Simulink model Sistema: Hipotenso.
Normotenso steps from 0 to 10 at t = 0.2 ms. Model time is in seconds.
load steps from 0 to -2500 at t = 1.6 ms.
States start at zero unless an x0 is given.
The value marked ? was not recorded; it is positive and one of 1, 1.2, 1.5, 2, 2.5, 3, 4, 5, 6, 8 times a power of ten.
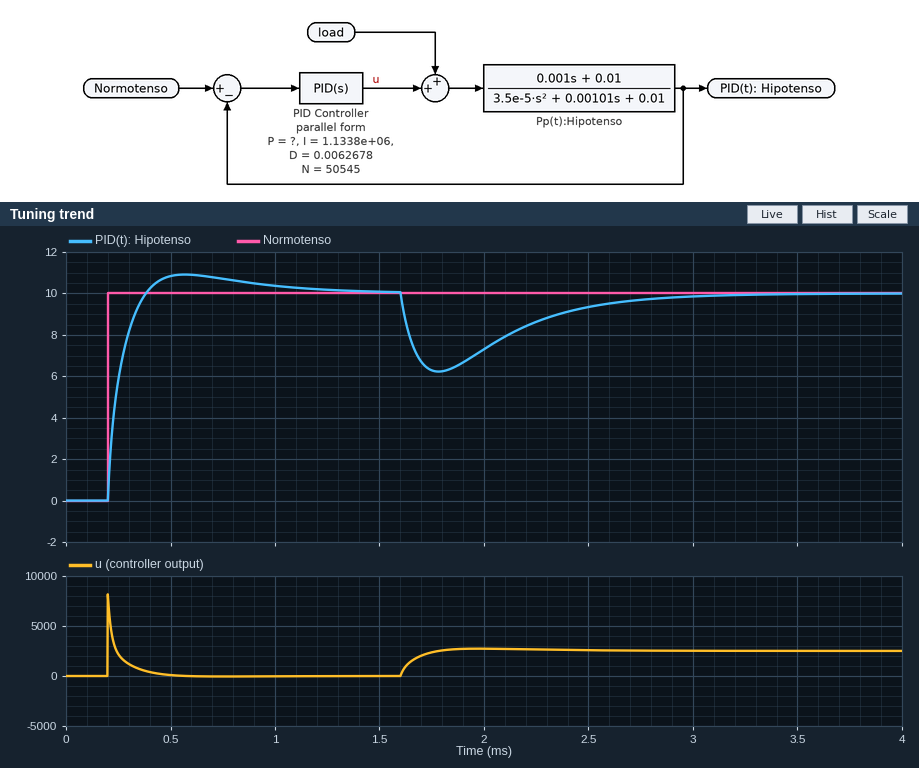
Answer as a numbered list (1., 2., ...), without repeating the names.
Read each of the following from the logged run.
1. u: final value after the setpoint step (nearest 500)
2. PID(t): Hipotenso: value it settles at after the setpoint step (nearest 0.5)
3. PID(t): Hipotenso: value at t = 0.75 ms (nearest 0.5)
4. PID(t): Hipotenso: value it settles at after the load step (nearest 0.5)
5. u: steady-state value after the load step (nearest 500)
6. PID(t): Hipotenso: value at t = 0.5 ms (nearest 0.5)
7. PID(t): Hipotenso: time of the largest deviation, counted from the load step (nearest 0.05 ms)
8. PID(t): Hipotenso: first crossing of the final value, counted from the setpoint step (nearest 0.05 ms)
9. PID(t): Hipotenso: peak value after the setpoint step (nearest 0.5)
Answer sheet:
1. 0
2. 10.0
3. 10.5
4. 10.0
5. 2500
6. 11.0
7. 0.20 ms
8. 0.20 ms
9. 11.0
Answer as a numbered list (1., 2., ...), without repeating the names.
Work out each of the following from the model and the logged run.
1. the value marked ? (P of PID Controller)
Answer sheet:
1. 500
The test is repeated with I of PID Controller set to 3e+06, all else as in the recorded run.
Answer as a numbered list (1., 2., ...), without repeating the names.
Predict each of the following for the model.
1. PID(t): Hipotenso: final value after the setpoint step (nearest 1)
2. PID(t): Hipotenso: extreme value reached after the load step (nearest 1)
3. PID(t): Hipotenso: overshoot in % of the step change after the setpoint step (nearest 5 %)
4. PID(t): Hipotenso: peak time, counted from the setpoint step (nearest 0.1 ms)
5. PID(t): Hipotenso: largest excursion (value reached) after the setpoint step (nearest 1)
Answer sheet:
1. 10
2. 7
3. 15 %
4. 0.3 ms
5. 12
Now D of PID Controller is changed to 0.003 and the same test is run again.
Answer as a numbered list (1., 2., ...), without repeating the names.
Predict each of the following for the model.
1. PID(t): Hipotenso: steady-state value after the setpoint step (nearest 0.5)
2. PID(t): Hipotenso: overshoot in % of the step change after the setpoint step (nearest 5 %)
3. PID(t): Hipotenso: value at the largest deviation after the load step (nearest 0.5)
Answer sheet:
1. 10.0
2. 10 %
3. 6.0
